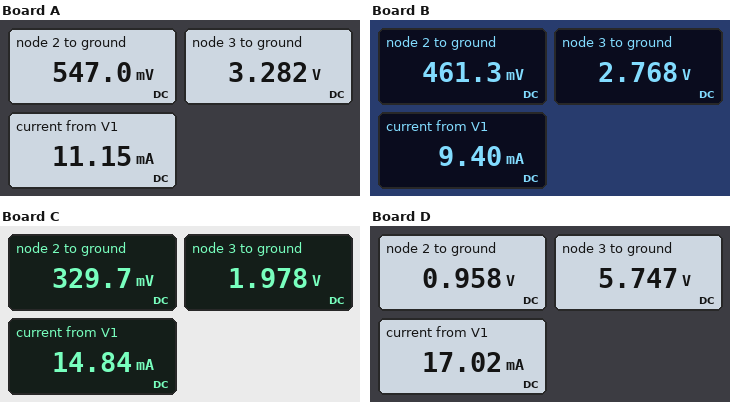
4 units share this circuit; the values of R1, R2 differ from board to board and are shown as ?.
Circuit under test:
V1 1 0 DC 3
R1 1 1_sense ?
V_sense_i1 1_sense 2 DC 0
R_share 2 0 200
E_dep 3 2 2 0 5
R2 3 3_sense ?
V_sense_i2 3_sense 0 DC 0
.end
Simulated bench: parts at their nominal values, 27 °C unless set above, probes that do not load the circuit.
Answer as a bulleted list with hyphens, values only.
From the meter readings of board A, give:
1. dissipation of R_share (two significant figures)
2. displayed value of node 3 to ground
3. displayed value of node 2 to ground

- 1.5 mW
- 3.282 V
- 547.0 mV
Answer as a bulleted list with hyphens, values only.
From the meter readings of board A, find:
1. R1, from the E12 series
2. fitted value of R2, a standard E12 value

- 220 Ω
- 390 Ω
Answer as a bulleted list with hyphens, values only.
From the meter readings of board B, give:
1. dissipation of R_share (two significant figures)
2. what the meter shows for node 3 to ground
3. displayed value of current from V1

- 1.1 mW
- 2.768 V
- 9.40 mA
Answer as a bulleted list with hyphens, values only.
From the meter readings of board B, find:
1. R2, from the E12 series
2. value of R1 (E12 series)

- 390 Ω
- 270 Ω
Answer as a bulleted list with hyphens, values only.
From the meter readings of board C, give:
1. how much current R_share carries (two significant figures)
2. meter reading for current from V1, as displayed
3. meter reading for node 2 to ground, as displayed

- 1.6 mA
- 14.84 mA
- 329.7 mV
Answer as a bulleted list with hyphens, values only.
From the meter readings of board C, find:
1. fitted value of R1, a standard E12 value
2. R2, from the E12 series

- 180 Ω
- 150 Ω
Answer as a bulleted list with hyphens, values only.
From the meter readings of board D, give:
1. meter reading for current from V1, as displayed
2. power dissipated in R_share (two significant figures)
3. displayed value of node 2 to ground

- 17.02 mA
- 4.6 mW
- 0.958 V
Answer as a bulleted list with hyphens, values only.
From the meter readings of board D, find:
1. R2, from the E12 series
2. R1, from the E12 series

- 470 Ω
- 120 Ω
